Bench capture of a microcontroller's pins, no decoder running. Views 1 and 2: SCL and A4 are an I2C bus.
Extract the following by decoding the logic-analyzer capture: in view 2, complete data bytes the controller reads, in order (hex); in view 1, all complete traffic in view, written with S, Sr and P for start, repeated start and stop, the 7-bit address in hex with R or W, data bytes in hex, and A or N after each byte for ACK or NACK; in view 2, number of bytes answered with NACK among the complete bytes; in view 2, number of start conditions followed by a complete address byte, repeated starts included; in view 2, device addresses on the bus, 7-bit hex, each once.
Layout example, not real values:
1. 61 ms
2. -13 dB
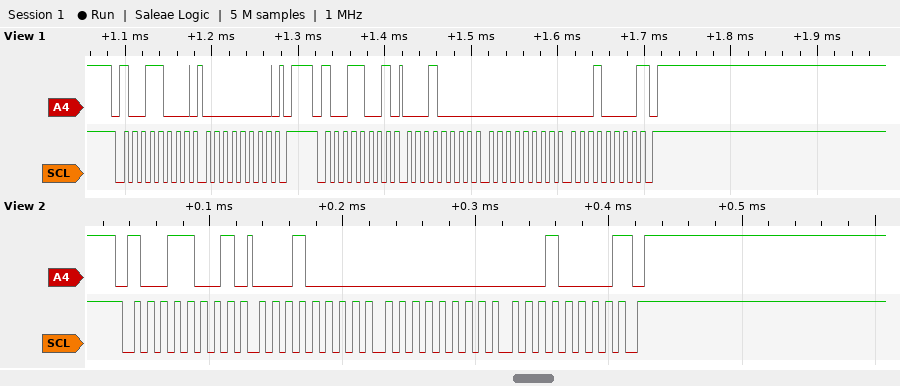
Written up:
1. 10 00 10
2. S 4CW A 00 A P S 4CR A 10 A 00 A 10 N P
3. 1
4. 1
5. 0x4C
